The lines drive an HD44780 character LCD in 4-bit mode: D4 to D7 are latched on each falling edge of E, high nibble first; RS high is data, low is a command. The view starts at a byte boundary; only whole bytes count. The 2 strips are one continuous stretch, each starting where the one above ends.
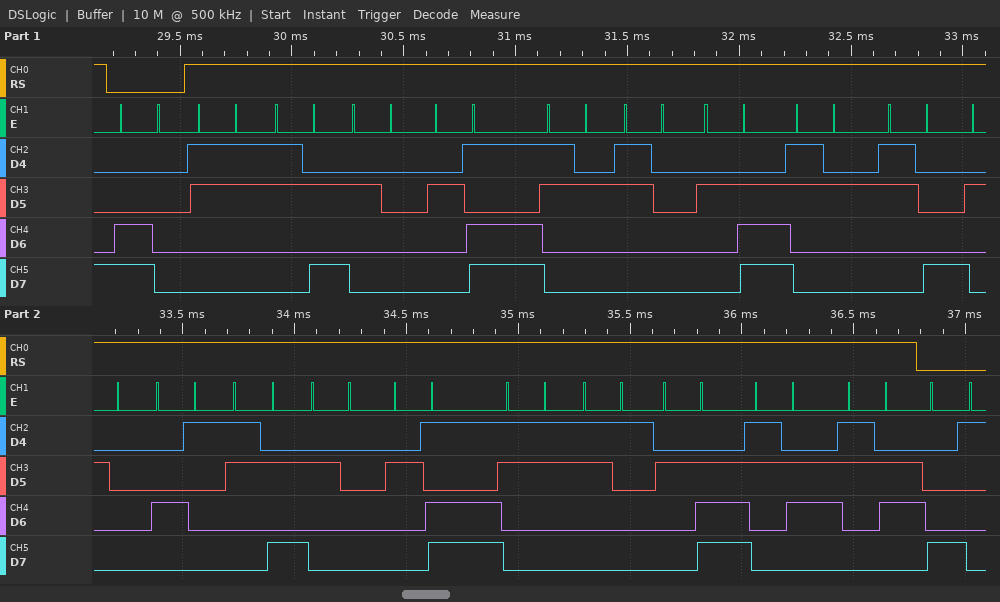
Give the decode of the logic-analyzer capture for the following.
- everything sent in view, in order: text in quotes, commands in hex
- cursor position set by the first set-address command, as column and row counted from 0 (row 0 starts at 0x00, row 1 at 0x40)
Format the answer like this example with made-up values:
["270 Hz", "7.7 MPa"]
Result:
["0xC0 \"3: -20.28 A: -31.66\" 0x81", "column 0, row 1"]
